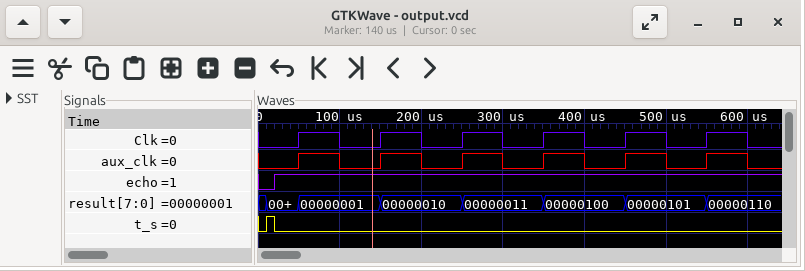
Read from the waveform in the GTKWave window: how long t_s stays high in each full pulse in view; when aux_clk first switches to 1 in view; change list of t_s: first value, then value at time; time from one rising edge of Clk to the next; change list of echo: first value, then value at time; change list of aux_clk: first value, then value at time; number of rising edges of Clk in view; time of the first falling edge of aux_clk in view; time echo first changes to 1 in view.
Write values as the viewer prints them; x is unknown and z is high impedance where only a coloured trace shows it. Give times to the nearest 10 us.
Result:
10 us
50 us
0, 1 at 10 us, 0 at 20 us
100 us
0, 1 at 20 us
0, 1 at 50 us, 0 at 100 us, 1 at 150 us, 0 at 200 us, 1 at 250 us, 0 at 300 us, 1 at 350 us, 0 at 400 us, 1 at 450 us, 0 at 500 us, 1 at 550 us, 0 at 600 us
6
100 us
20 us
